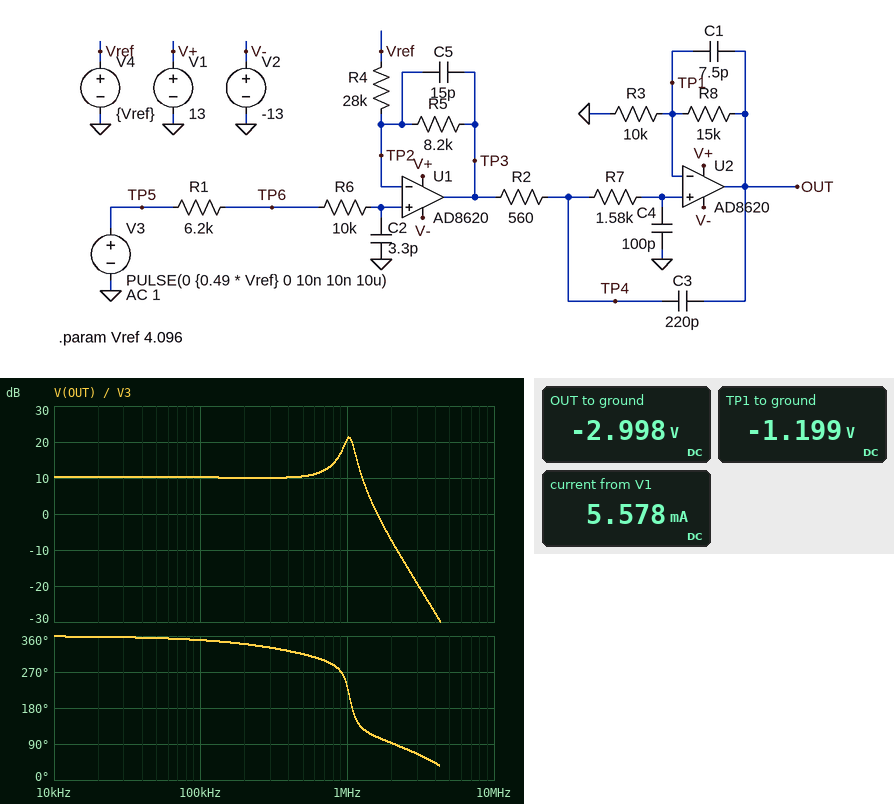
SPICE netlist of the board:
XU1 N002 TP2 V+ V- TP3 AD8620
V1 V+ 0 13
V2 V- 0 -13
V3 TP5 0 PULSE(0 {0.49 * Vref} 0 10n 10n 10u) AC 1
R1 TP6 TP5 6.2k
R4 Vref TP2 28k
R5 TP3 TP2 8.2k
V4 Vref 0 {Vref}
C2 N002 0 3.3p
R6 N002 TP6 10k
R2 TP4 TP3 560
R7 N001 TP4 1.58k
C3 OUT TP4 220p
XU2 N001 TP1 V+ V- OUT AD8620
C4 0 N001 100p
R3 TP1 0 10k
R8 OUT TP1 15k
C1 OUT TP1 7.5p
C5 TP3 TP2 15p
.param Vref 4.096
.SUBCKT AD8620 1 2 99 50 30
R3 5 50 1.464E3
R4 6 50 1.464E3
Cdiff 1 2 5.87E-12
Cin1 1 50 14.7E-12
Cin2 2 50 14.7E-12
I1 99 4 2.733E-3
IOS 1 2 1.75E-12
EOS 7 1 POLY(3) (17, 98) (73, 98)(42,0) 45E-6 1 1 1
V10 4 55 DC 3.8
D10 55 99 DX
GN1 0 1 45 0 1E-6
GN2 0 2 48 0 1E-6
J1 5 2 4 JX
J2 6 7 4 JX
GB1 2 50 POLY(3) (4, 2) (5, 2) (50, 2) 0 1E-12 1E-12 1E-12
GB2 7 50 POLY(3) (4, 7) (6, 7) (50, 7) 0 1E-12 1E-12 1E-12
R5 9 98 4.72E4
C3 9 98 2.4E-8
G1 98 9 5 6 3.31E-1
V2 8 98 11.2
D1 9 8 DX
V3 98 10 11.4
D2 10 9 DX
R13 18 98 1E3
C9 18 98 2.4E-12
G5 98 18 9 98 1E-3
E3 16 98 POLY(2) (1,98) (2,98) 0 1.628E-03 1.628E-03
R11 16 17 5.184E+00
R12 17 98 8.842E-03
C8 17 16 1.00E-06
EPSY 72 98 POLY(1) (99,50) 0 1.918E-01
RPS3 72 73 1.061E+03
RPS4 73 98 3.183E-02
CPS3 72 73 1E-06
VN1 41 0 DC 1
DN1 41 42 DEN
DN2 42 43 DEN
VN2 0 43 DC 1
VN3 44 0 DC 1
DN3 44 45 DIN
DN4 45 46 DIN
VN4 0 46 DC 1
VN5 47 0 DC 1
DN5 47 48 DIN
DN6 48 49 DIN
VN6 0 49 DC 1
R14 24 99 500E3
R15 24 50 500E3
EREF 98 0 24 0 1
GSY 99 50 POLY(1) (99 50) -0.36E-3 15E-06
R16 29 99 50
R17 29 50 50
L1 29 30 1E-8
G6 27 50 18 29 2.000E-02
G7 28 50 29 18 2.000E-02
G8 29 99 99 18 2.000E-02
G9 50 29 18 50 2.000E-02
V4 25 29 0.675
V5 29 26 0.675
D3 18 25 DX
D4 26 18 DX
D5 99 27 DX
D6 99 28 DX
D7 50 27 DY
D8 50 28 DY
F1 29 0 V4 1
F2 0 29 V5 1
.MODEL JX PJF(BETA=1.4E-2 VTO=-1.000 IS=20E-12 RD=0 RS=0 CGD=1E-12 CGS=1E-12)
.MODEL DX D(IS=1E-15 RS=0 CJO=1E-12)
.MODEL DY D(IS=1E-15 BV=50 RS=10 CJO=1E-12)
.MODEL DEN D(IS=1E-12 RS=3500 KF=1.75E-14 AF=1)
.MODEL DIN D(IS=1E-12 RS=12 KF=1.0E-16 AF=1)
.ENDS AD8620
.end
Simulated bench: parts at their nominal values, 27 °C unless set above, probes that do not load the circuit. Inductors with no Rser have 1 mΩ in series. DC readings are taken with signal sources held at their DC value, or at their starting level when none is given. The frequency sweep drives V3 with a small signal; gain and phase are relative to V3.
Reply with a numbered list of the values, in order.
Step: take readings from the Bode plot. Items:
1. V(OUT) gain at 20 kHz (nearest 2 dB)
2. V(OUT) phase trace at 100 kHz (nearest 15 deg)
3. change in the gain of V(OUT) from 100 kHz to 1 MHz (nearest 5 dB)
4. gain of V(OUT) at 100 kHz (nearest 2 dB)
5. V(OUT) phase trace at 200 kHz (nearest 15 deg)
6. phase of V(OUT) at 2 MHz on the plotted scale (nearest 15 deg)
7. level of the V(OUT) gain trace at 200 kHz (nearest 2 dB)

1. 10 dB
2. 345 deg
3. 10 dB
4. 10 dB
5. 345 deg
6. 90 deg
7. 10 dB
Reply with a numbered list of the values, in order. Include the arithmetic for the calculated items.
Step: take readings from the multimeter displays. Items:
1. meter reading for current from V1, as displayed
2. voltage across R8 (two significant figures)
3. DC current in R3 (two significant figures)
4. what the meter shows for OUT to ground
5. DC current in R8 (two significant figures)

1. 5.578 mA
2. -1.199 V - (-2.998 V) = 1.8 V
3. (0 V - (-1.199 V)) / 10 kΩ = 120 µA
4. -2.998 V
5. (-1.199 V - (-2.998 V)) / 15 kΩ = 120 µA
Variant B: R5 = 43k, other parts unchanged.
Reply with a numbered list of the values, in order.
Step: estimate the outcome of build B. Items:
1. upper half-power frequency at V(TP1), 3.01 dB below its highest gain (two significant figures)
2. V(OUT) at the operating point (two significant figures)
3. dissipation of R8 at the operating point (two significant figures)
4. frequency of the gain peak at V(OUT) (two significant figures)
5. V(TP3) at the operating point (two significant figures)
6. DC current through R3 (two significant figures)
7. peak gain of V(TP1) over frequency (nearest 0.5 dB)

1. 790 kHz
2. -12 V
3. 3.6 mW
4. 660 kHz
5. -6.3 V
6. 490 µA
7. -18.0 dB
